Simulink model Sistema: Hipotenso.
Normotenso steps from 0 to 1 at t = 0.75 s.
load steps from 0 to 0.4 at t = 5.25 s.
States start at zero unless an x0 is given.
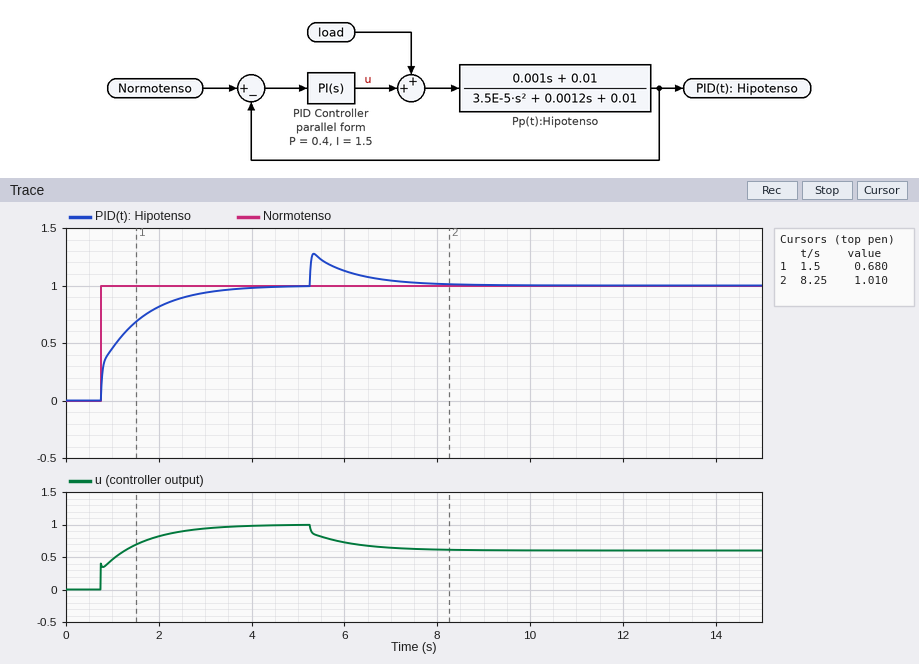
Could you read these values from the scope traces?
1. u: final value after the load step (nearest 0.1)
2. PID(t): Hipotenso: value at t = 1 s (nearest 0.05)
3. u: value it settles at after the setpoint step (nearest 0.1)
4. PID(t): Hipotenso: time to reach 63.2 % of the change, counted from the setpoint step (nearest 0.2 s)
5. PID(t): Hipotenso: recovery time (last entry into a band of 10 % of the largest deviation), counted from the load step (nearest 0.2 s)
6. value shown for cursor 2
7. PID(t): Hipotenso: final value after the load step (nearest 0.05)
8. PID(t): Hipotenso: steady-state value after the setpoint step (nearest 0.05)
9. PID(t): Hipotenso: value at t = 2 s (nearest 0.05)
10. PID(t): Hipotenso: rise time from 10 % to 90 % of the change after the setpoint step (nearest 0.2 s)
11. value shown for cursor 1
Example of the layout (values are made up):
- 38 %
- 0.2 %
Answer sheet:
- 0.6
- 0.45
- 1.0
- 0.6 s
- 2.2 s
- 1.010
- 1.00
- 1.00
- 0.80
- 1.8 s
- 0.680
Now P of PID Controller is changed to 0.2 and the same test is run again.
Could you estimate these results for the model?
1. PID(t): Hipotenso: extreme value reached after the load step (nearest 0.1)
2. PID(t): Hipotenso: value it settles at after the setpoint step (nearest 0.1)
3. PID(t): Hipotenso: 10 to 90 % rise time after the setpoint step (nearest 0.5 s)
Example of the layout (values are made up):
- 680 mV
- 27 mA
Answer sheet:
- 1.3
- 1.0
- 1.5 s
